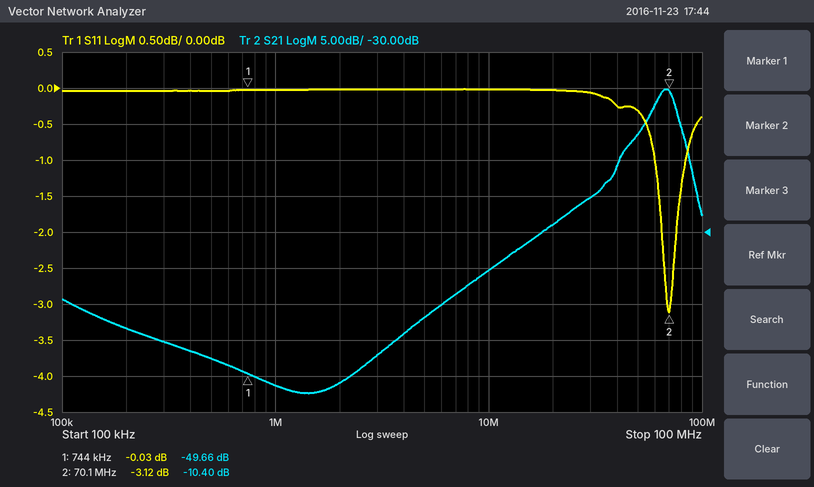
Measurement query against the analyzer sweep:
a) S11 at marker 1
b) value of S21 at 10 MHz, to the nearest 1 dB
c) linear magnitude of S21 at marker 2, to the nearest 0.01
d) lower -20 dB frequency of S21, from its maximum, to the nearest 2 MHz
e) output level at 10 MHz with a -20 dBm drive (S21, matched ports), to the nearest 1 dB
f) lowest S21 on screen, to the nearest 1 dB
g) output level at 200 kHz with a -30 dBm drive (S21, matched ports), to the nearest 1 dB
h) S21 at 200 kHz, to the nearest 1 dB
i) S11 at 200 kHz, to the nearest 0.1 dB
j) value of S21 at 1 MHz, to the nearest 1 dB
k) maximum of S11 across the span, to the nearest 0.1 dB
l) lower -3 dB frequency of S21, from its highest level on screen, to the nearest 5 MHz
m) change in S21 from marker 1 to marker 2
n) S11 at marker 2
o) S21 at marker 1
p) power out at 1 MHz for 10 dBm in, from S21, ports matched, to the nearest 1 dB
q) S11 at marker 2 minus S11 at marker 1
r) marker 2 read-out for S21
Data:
-0.03 dB
-35 dB
0.30
18 MHz
-55 dBm
-52 dB
-73 dBm
-43 dB
0.0 dB
-51 dB
0.0 dB
60 MHz
39.26 dB
-3.12 dB
-49.66 dB
-41 dBm
-3.09 dB
-10.40 dB
